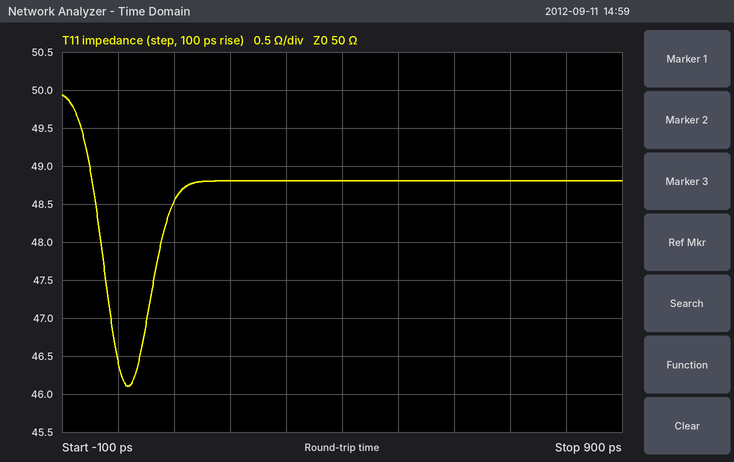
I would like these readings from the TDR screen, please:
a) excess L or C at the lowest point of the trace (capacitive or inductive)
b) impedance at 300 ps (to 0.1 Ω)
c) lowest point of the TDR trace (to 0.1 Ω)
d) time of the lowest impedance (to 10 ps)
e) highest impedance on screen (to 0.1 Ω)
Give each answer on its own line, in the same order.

capacitive
48.8 Ω
46.1 Ω
20 ps
49.9 Ω
